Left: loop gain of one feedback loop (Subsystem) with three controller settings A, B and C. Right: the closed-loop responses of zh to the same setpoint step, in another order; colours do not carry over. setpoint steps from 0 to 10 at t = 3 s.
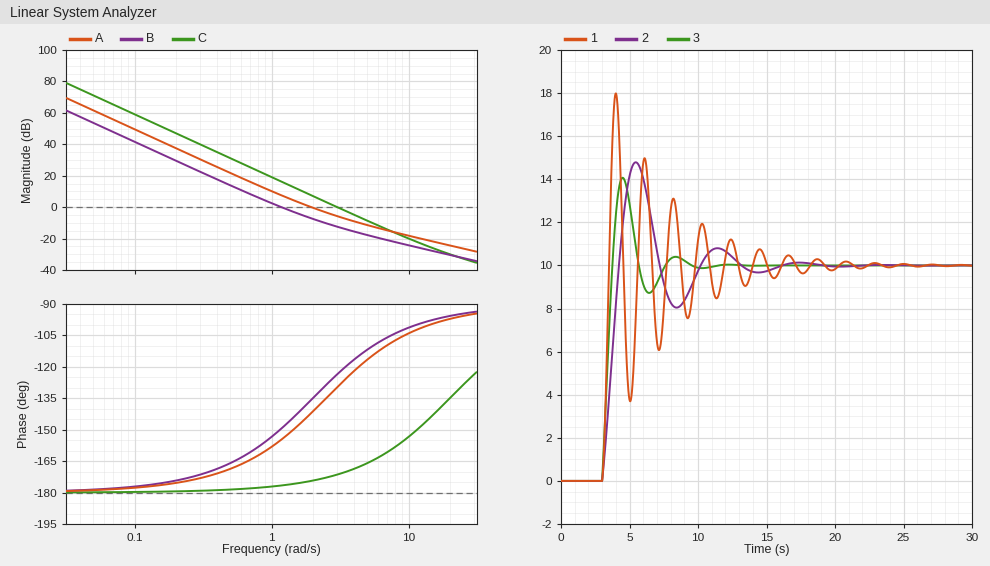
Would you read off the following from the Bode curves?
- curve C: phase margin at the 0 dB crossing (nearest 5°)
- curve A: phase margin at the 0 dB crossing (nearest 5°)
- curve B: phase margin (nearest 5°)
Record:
10°
40°
30°
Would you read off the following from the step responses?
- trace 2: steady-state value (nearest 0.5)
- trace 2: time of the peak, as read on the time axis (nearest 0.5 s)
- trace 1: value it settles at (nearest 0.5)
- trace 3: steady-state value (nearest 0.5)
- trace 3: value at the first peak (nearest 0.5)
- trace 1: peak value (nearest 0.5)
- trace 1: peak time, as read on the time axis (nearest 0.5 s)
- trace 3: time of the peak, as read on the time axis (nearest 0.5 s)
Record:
10.0
5.5 s
10.0
10.0
14.0
18.0
4.0 s
4.5 s
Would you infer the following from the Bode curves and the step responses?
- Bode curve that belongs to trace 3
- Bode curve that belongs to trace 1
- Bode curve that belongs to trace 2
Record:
A
C
B
